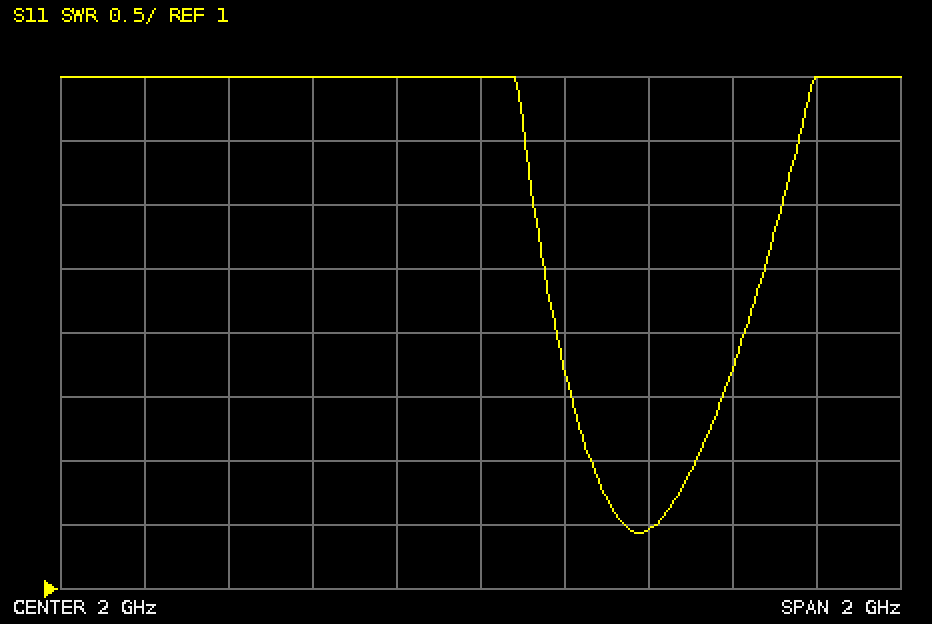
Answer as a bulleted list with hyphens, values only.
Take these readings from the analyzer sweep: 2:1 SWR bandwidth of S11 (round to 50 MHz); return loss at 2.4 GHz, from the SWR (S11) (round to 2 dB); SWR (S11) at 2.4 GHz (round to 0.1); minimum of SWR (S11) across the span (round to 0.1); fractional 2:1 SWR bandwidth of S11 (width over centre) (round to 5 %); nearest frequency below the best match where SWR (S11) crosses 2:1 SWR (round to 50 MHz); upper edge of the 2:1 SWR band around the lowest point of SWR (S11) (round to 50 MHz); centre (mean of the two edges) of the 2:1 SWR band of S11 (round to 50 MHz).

- 250 MHz
- 14 dB
- 1.5
- 1.4
- 10 %
- 2.25 GHz
- 2.50 GHz
- 2.40 GHz
